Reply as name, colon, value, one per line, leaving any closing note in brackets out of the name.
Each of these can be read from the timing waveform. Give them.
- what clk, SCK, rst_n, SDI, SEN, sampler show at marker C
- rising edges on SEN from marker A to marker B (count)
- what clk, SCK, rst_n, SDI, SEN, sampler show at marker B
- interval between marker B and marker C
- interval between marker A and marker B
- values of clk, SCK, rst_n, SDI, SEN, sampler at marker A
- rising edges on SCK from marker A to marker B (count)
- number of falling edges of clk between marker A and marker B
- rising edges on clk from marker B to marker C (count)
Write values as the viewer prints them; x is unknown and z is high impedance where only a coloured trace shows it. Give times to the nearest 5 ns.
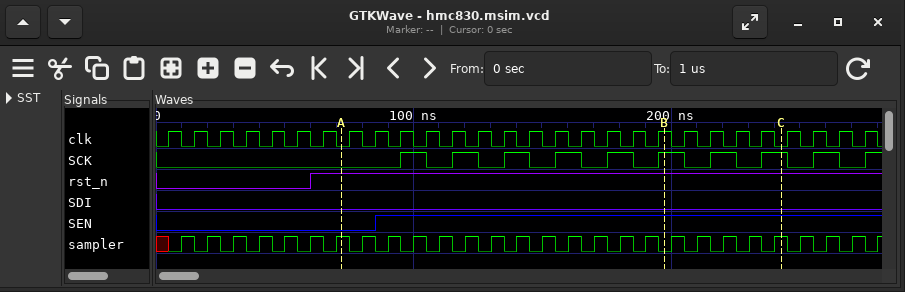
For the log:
what clk, SCK, rst_n, SDI, SEN, sampler show at marker C: clk=0, SCK=1, rst_n=1, SDI=0, SEN=1, sampler=1
rising edges on SEN from marker A to marker B: 1
what clk, SCK, rst_n, SDI, SEN, sampler show at marker B: clk=1, SCK=1, rst_n=1, SDI=0, SEN=1, sampler=0
interval between marker B and marker C: 45 ns
interval between marker A and marker B: 125 ns
values of clk, SCK, rst_n, SDI, SEN, sampler at marker A: clk=0, SCK=0, rst_n=1, SDI=0, SEN=0, sampler=1
rising edges on SCK from marker A to marker B: 6
number of falling edges of clk between marker A and marker B: 12
rising edges on clk from marker B to marker C: 4
